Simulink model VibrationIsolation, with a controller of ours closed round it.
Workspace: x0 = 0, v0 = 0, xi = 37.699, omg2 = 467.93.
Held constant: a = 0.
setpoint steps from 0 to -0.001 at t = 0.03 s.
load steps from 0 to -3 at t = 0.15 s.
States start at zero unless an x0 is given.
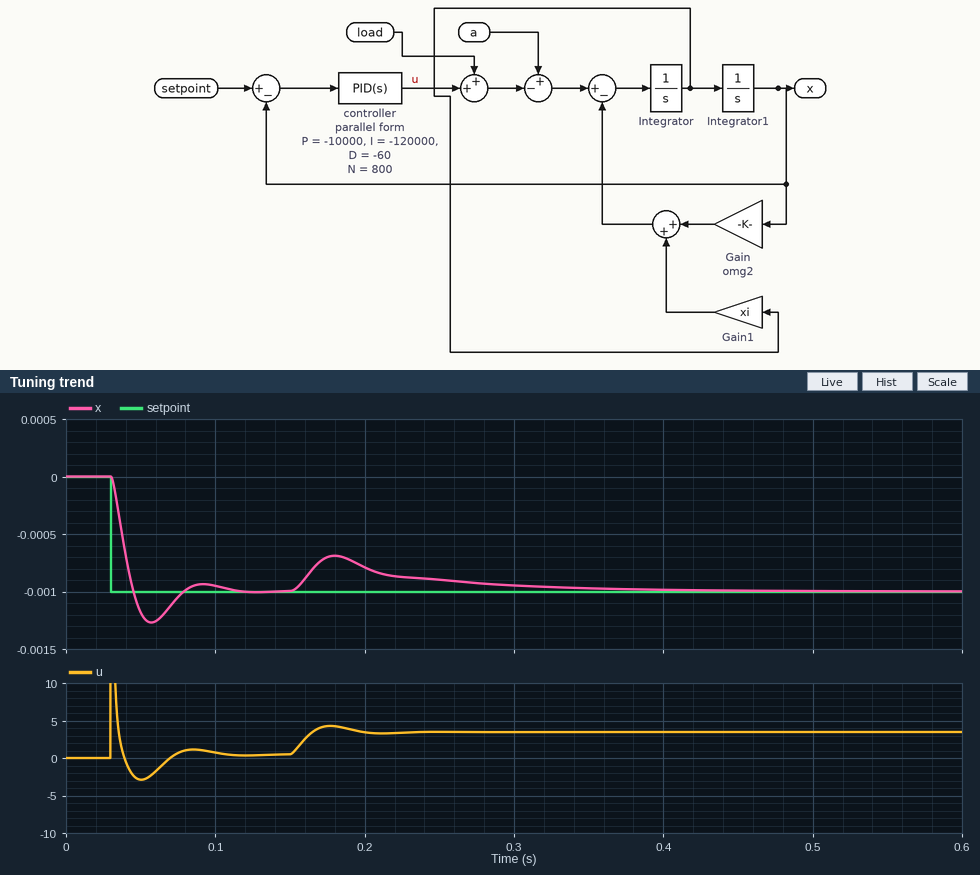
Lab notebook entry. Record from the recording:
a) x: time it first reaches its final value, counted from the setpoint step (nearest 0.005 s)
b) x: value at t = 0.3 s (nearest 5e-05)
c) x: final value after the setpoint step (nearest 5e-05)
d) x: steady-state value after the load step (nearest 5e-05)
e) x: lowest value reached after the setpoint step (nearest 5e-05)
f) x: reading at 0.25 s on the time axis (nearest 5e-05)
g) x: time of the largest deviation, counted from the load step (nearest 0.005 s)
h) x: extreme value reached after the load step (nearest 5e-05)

0.015 s
-0.00095
-0.00100
-0.00100
-0.00125
-0.00090
0.030 s
-0.00070
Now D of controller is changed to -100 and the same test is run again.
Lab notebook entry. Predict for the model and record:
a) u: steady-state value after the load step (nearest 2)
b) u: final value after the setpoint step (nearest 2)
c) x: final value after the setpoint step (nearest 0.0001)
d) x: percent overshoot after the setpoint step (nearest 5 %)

4
0
-0.0010
15 %
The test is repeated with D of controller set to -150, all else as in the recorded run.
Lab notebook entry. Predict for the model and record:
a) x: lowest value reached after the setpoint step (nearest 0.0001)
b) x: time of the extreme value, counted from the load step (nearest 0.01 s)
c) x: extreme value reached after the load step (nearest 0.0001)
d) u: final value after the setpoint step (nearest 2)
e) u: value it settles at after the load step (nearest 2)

-0.0011
0.04 s
-0.0008
0
4
